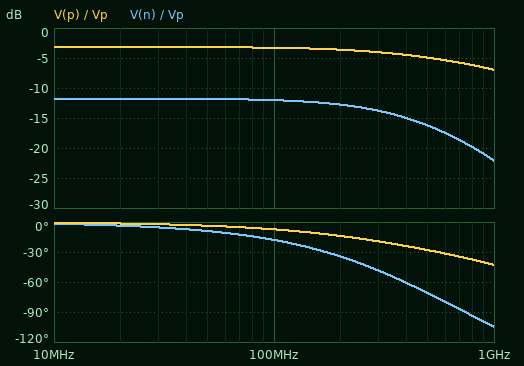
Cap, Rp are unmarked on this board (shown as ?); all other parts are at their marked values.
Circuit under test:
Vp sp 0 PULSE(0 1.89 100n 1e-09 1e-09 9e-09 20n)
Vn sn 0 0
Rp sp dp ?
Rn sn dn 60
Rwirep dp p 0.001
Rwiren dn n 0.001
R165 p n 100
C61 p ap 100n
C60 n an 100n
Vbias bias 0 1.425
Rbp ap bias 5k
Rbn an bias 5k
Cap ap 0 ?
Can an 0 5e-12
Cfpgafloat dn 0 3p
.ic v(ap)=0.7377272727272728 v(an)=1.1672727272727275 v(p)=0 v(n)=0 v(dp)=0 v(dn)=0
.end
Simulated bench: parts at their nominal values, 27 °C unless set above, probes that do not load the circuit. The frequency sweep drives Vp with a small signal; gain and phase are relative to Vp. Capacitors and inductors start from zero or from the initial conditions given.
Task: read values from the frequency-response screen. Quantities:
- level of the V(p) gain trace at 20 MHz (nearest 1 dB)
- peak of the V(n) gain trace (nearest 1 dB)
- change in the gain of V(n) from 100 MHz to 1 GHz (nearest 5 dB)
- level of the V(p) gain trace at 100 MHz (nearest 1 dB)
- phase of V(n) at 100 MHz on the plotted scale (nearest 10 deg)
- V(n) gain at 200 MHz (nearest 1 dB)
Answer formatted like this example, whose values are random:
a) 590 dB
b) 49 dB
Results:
a) -3 dB
b) -12 dB
c) -10 dB
d) -3 dB
e) -20 deg
f) -13 dB
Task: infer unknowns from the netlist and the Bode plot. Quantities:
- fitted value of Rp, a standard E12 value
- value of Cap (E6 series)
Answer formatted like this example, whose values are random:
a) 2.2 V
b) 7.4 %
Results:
a) 68 Ω
b) 3.3 pF
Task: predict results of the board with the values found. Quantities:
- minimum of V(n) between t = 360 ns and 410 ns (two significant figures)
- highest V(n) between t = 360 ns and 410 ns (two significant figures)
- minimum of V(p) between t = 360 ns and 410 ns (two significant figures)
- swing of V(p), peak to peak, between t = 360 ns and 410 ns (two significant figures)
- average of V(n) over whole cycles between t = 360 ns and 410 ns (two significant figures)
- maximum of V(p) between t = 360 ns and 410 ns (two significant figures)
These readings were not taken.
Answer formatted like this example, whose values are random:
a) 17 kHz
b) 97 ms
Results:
a) 4.7 mV
b) 490 mV
c) 7.4 mV
d) 1.3 V
e) 250 mV
f) 1.3 V
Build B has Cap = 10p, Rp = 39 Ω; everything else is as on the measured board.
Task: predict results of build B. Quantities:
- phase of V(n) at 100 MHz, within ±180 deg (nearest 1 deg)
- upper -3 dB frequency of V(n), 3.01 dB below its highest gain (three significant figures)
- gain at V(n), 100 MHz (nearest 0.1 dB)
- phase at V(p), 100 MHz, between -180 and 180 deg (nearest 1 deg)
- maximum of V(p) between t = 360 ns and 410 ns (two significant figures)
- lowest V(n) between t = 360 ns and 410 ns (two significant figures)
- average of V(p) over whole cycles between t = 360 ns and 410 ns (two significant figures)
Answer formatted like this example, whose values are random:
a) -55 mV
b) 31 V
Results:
a) -23 deg
b) 311 MHz
c) -10.9 dB
d) -12 deg
e) 1.5 V
f) 3.7 mV
g) 760 mV
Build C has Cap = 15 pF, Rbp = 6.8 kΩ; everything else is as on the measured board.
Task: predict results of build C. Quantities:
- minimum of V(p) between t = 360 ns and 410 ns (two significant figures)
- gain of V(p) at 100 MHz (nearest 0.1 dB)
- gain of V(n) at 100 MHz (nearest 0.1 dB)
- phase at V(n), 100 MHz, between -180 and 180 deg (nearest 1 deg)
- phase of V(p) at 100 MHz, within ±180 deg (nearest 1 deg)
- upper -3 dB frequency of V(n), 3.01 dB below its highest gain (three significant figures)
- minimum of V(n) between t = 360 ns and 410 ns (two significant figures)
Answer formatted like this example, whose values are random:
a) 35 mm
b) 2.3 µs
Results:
a) 5.7 mV
b) -4.1 dB
c) -12.8 dB
d) -36 deg
e) -25 deg
f) 183 MHz
g) 4.0 mV
